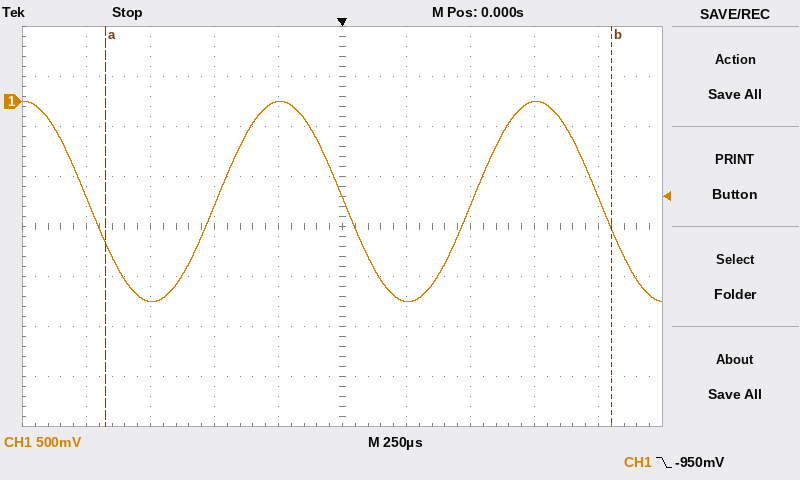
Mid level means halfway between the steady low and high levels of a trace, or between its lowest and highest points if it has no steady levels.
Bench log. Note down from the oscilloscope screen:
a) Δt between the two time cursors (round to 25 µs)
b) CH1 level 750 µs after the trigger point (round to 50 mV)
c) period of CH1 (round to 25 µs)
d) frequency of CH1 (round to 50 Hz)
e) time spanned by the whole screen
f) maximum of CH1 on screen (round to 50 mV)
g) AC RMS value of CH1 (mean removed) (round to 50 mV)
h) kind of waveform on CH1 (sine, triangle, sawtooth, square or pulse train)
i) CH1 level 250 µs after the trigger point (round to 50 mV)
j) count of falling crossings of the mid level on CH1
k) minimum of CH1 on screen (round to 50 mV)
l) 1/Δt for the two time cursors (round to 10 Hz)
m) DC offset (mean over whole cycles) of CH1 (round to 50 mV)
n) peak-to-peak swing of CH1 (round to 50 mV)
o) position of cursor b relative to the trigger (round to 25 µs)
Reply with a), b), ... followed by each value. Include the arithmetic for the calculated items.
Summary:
a) 1.975 ms
b) 0 mV
c) 1.000 ms
d) 1 / 1.000 ms ≈ 1.00 kHz
e) 2.5 ms
f) 0 mV
g) 2.00 V / (2√2) ≈ 707 mV, so 700 mV to the nearest 50 mV
h) sine
i) -2.00 V
j) 3
k) -2.00 V
l) 1 / 1.975 ms ≈ 510 Hz
m) (0 mV + (-2.00 V)) / 2 ≈ -1.00 V
n) 0 mV − (-2.00 V) = 2.00 V
o) +1.050 ms
